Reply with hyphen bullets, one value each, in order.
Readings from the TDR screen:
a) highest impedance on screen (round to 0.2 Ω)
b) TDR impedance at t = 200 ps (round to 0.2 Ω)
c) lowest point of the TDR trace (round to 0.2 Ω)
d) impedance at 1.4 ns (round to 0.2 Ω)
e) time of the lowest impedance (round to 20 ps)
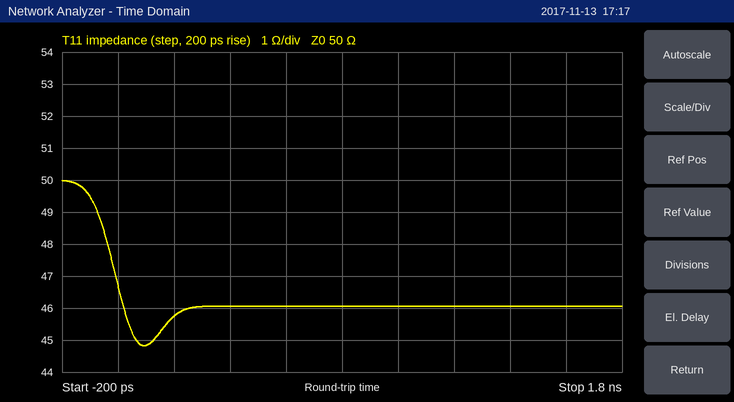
- 50.0 Ω
- 45.8 Ω
- 44.8 Ω
- 46.0 Ω
- 100 ps
